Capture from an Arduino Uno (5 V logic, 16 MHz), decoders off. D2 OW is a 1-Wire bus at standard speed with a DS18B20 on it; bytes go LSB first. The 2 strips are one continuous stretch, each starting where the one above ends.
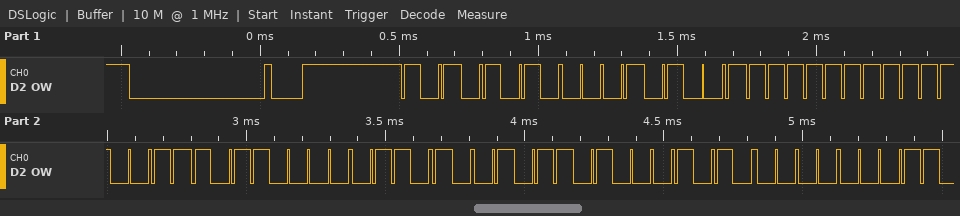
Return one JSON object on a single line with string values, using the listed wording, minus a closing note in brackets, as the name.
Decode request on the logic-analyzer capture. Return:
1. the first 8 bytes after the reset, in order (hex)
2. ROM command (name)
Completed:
{"the first 8 bytes after the reset, in order": "55 28 FF CF 0D 96 16 05", "ROM command": "Match ROM"}
